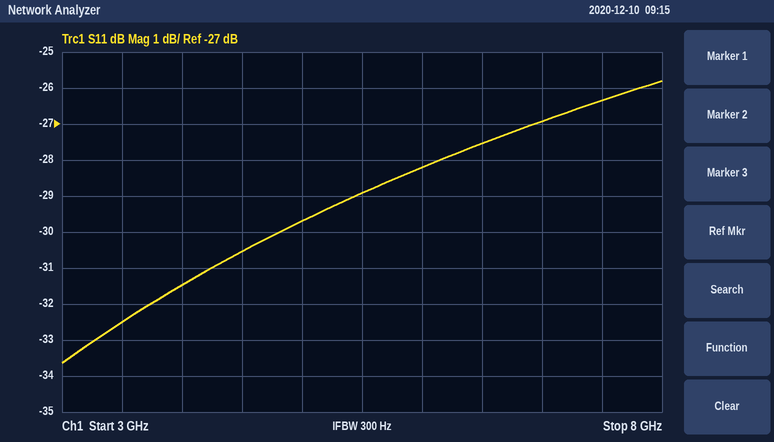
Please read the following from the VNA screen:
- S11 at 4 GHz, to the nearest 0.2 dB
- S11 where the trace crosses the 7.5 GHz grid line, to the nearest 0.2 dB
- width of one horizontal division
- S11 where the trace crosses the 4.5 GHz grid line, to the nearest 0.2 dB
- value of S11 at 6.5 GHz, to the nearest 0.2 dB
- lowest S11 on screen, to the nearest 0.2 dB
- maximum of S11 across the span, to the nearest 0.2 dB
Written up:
-31.4 dB
-26.4 dB
500 MHz
-30.6 dB
-27.6 dB
-33.6 dB
-25.8 dB
